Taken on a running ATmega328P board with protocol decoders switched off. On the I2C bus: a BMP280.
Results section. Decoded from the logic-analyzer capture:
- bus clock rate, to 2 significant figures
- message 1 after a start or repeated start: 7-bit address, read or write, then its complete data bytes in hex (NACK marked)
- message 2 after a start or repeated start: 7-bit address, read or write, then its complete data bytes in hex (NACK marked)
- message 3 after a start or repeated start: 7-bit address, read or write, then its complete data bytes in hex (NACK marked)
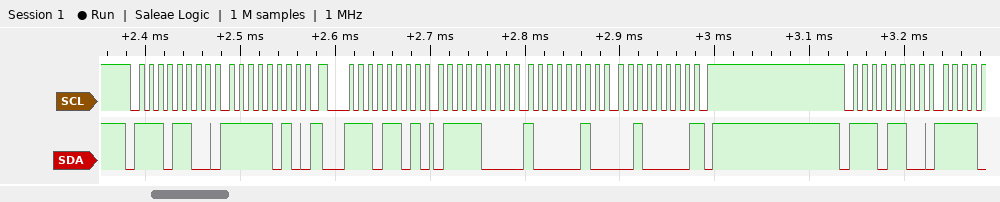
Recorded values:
100 kHz
0x76 write: FA
0x76 read: 78 82 20 NACK
0x76 write
